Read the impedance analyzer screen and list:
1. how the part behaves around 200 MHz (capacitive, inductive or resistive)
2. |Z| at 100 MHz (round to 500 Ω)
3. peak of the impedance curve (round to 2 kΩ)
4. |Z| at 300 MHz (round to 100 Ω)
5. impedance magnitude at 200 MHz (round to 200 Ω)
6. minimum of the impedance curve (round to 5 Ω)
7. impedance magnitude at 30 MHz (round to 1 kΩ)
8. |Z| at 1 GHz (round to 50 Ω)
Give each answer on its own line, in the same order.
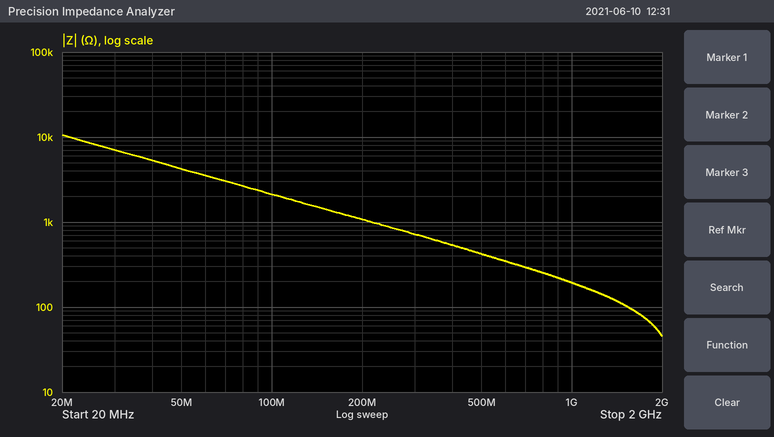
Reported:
capacitive
2.0 kΩ
10 kΩ
700 Ω
1.0 kΩ
45 Ω
7 kΩ
200 Ω
